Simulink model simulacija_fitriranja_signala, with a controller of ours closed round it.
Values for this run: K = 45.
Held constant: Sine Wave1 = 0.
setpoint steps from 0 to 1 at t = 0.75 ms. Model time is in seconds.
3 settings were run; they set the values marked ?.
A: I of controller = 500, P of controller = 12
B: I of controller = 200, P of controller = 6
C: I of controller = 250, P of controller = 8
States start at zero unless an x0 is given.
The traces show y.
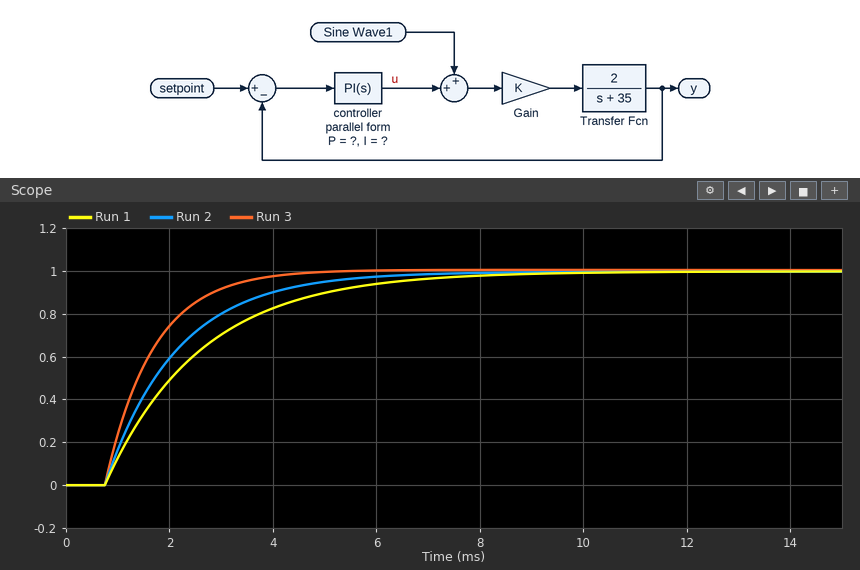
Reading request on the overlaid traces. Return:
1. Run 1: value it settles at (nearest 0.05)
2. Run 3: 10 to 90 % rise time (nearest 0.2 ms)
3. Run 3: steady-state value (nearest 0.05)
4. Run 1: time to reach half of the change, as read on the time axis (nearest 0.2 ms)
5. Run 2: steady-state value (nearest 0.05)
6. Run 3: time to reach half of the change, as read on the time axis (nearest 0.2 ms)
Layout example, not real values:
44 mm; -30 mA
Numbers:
1.00; 2.0 ms; 1.00; 2.0 ms; 1.00; 1.4 ms
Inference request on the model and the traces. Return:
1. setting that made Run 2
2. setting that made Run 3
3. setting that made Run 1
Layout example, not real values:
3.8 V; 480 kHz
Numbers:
C; A; B
